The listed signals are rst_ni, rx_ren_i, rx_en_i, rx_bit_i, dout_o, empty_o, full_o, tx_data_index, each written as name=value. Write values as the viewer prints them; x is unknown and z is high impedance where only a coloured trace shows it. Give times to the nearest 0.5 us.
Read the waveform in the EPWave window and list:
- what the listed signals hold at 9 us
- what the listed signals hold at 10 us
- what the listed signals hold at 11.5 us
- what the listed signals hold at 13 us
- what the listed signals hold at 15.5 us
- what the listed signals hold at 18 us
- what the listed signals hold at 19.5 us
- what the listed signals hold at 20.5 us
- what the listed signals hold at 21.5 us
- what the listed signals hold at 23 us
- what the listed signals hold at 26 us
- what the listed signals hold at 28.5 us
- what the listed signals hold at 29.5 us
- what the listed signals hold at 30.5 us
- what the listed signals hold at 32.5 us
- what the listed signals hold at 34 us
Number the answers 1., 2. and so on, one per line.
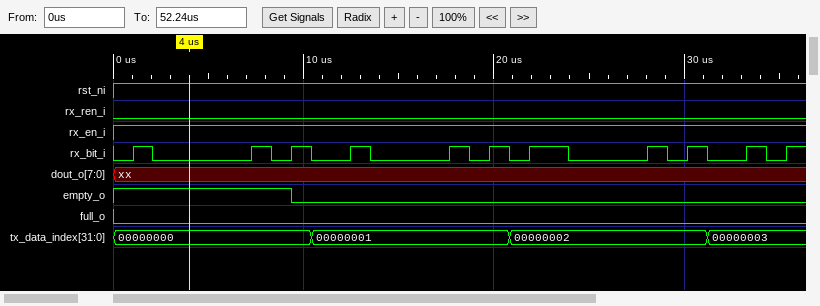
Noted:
1. rst_ni=1, rx_ren_i=0, rx_en_i=1, rx_bit_i=0, dout_o=xx, empty_o=1, full_o=0, tx_data_index=00000000
2. rst_ni=1, rx_ren_i=0, rx_en_i=1, rx_bit_i=1, dout_o=xx, empty_o=0, full_o=0, tx_data_index=00000000
3. rst_ni=1, rx_ren_i=0, rx_en_i=1, rx_bit_i=0, dout_o=xx, empty_o=0, full_o=0, tx_data_index=00000001
4. rst_ni=1, rx_ren_i=0, rx_en_i=1, rx_bit_i=1, dout_o=xx, empty_o=0, full_o=0, tx_data_index=00000001
5. rst_ni=1, rx_ren_i=0, rx_en_i=1, rx_bit_i=0, dout_o=xx, empty_o=0, full_o=0, tx_data_index=00000001
6. rst_ni=1, rx_ren_i=0, rx_en_i=1, rx_bit_i=1, dout_o=xx, empty_o=0, full_o=0, tx_data_index=00000001
7. rst_ni=1, rx_ren_i=0, rx_en_i=1, rx_bit_i=0, dout_o=xx, empty_o=0, full_o=0, tx_data_index=00000001
8. rst_ni=1, rx_ren_i=0, rx_en_i=1, rx_bit_i=1, dout_o=xx, empty_o=0, full_o=0, tx_data_index=00000001
9. rst_ni=1, rx_ren_i=0, rx_en_i=1, rx_bit_i=0, dout_o=xx, empty_o=0, full_o=0, tx_data_index=00000002
10. rst_ni=1, rx_ren_i=0, rx_en_i=1, rx_bit_i=1, dout_o=xx, empty_o=0, full_o=0, tx_data_index=00000002
11. rst_ni=1, rx_ren_i=0, rx_en_i=1, rx_bit_i=0, dout_o=xx, empty_o=0, full_o=0, tx_data_index=00000002
12. rst_ni=1, rx_ren_i=0, rx_en_i=1, rx_bit_i=1, dout_o=xx, empty_o=0, full_o=0, tx_data_index=00000002
13. rst_ni=1, rx_ren_i=0, rx_en_i=1, rx_bit_i=0, dout_o=xx, empty_o=0, full_o=0, tx_data_index=00000002
14. rst_ni=1, rx_ren_i=0, rx_en_i=1, rx_bit_i=1, dout_o=xx, empty_o=0, full_o=0, tx_data_index=00000002
15. rst_ni=1, rx_ren_i=0, rx_en_i=1, rx_bit_i=0, dout_o=xx, empty_o=0, full_o=0, tx_data_index=00000003
16. rst_ni=1, rx_ren_i=0, rx_en_i=1, rx_bit_i=1, dout_o=xx, empty_o=0, full_o=0, tx_data_index=00000003
